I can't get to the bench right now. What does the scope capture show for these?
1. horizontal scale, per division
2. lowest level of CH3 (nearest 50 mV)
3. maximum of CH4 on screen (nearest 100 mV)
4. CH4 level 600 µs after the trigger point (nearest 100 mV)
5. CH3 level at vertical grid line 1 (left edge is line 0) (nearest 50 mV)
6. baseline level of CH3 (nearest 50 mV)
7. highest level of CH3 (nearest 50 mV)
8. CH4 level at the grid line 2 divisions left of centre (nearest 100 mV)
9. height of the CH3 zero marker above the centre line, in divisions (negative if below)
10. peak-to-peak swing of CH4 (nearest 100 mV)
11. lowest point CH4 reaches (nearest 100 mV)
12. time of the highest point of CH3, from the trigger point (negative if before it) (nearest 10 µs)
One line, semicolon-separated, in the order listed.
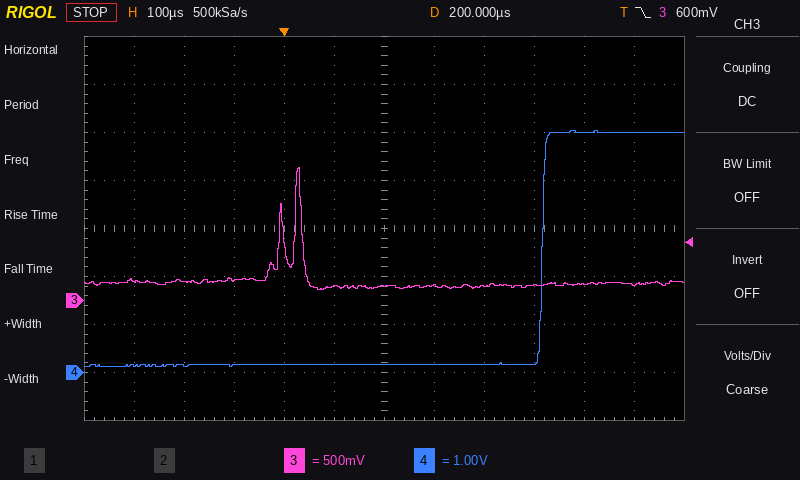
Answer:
100 µs; 100 mV; 5.0 V; 5.0 V; 200 mV; 150 mV; 1.40 V; 200 mV; -1.5 div; 4.9 V; 100 mV; +30 µs
